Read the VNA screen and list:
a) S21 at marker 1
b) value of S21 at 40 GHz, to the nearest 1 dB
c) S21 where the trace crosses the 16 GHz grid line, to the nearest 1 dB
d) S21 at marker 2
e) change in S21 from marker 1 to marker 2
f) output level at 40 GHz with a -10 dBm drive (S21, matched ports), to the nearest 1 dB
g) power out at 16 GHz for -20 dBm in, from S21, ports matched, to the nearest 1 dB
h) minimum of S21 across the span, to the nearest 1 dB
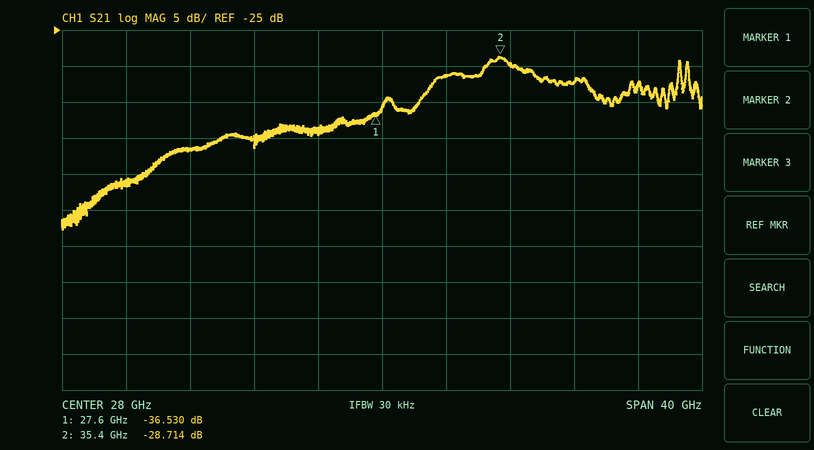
-36.530 dB
-32 dB
-42 dB
-28.714 dB
7.816 dB
-42 dBm
-62 dBm
-53 dB
